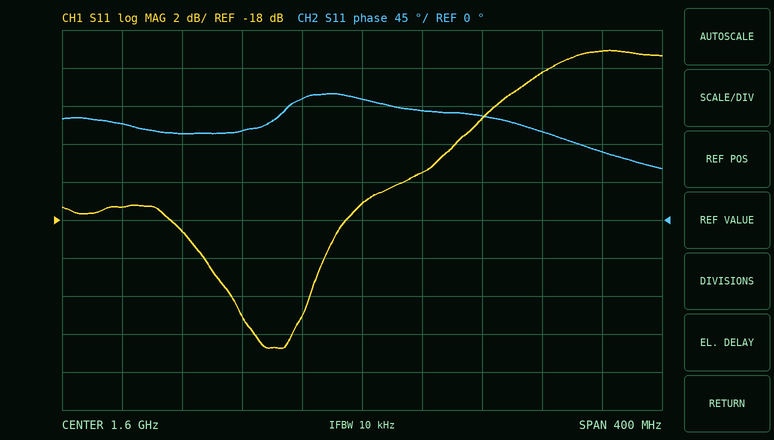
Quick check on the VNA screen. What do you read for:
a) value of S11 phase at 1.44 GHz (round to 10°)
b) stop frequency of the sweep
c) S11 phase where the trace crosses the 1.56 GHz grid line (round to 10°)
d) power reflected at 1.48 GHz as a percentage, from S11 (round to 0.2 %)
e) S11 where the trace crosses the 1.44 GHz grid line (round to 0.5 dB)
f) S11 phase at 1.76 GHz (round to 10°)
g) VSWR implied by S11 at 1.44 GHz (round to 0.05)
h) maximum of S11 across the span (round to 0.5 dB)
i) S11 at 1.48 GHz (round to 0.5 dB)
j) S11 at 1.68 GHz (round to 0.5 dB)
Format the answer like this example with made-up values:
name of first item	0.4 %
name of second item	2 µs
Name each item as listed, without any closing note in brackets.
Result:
value of S11 phase at 1.44 GHz	110°
stop frequency of the sweep	1.8 GHz
S11 phase where the trace crosses the 1.56 GHz grid line	140°
power reflected at 1.48 GHz as a percentage, from S11	1.4 %
S11 where the trace crosses the 1.44 GHz grid line	-17.5 dB
S11 phase at 1.76 GHz	80°
VSWR implied by S11 at 1.44 GHz	1.30
maximum of S11 across the span	-9.0 dB
S11 at 1.48 GHz	-18.5 dB
S11 at 1.68 GHz	-12.5 dB
